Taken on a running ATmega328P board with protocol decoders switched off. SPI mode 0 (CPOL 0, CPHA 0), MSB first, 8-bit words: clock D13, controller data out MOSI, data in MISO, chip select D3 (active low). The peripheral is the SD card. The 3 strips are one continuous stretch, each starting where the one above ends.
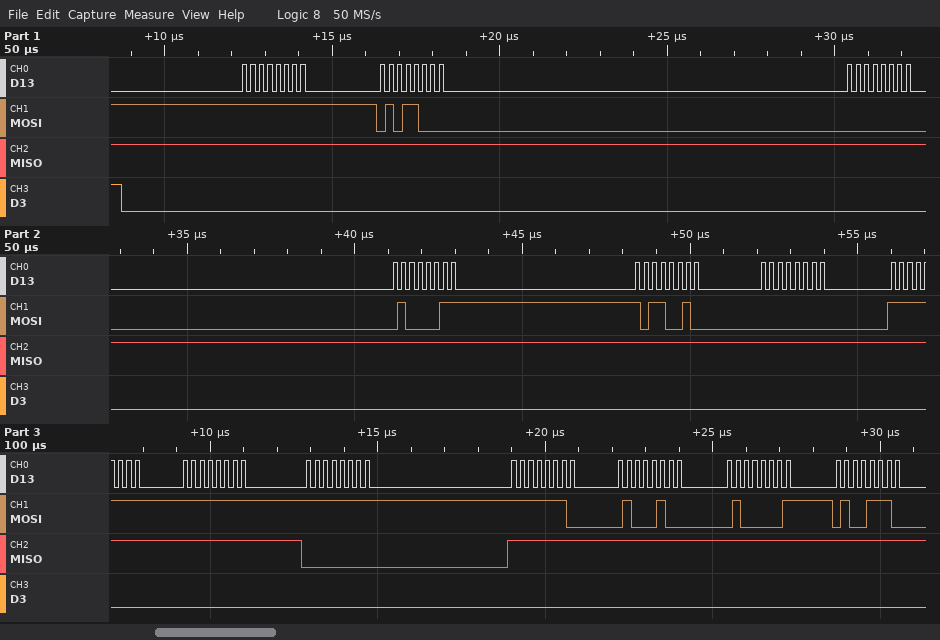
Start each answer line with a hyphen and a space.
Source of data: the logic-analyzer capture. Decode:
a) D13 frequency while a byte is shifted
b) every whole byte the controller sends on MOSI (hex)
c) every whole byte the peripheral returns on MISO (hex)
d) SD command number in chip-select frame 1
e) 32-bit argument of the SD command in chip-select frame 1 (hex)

- 4 MHz
- FF 58 00 43 B2 00 FF FF FF FE 44 41 4E
- FF FF FF FF FF FF FF FF 00 FF FF FF FF
- CMD24
- 0x0043B200
